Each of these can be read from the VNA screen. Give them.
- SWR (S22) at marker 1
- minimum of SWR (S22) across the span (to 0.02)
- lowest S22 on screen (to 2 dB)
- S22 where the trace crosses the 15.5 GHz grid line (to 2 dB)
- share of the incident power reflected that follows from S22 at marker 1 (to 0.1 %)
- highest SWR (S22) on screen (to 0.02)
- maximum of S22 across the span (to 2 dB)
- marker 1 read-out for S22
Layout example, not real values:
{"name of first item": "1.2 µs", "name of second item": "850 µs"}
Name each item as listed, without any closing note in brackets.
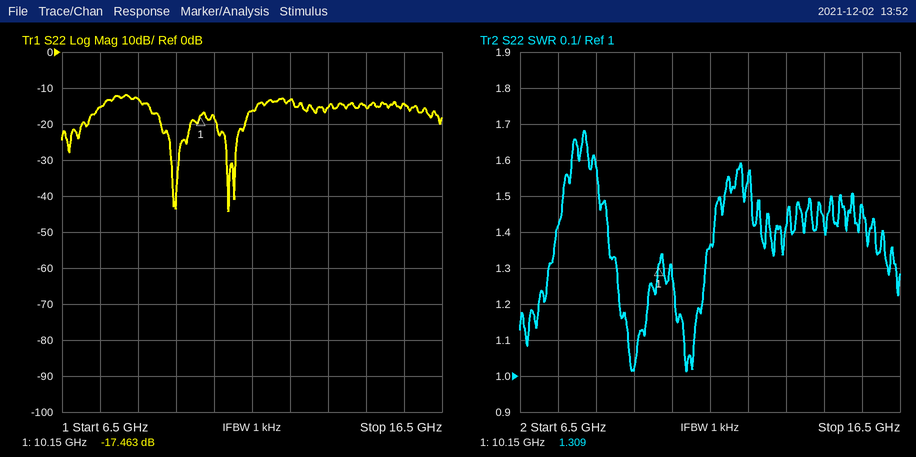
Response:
{"SWR (S22) at marker 1": "1.309", "minimum of SWR (S22) across the span": "1.02", "lowest S22 on screen": "-44 dB", "S22 where the trace crosses the 15.5 GHz grid line": "-14 dB", "share of the incident power reflected that follows from S22 at marker 1": "1.8 %", "highest SWR (S22) on screen": "1.68", "maximum of S22 across the span": "-12 dB", "marker 1 read-out for S22": "-17.463 dB"}
